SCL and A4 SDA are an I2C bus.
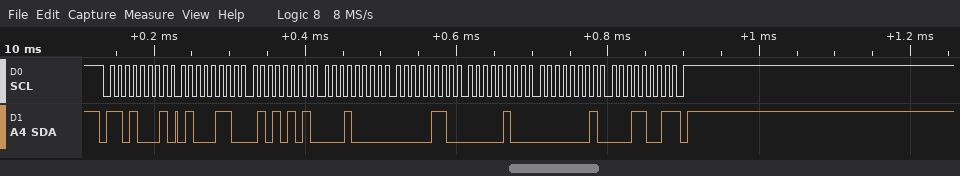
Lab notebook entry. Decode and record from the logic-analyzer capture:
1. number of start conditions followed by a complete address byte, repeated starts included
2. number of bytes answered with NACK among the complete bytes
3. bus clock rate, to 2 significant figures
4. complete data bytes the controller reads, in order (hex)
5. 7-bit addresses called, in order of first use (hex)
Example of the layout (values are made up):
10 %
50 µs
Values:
1
1
100 kHz
46 55 10 06 04 01 19
0x68
